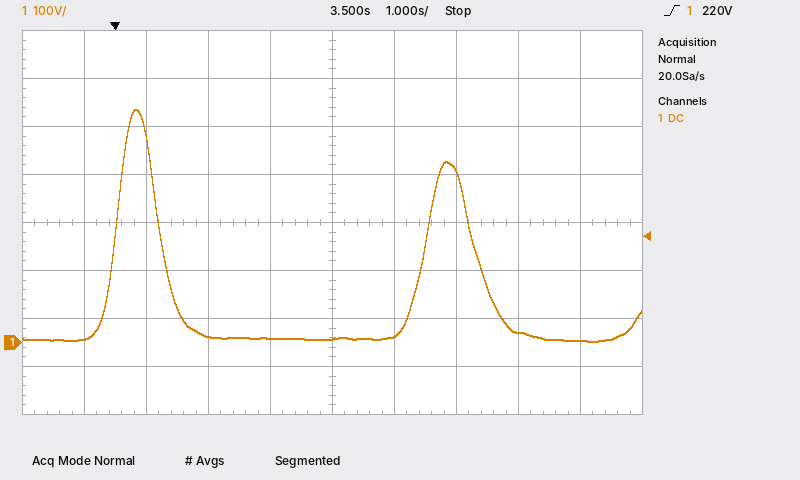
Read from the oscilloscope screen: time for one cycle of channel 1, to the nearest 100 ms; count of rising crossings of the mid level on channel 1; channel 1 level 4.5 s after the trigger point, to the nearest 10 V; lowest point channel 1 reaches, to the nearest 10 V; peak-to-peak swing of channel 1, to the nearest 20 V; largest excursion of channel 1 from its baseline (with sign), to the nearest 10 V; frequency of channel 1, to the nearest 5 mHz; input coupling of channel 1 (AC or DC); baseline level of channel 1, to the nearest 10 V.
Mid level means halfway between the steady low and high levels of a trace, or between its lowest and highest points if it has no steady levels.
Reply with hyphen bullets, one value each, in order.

- 5.0 s
- 2
- 10 V
- 0 V
- 480 V
- +480 V
- 200 mHz
- DC
- 10 V
